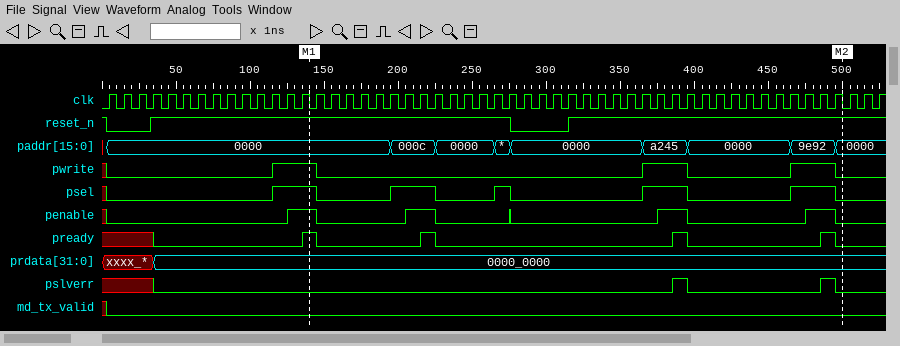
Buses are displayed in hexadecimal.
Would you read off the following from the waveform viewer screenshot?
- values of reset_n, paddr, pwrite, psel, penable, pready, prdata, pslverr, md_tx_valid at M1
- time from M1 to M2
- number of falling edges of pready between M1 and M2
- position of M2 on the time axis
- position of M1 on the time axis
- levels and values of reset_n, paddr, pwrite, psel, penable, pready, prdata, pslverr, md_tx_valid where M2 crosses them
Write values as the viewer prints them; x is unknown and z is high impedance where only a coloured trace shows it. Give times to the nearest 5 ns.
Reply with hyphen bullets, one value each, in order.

- reset_n=1, paddr=0000, pwrite=1, psel=1, penable=1, pready=1, prdata=0000_0000, pslverr=0, md_tx_valid=0
- 360 ns
- 4
- 500 ns
- 140 ns
- reset_n=1, paddr=0000, pwrite=0, psel=0, penable=0, pready=0, prdata=0000_0000, pslverr=0, md_tx_valid=0
